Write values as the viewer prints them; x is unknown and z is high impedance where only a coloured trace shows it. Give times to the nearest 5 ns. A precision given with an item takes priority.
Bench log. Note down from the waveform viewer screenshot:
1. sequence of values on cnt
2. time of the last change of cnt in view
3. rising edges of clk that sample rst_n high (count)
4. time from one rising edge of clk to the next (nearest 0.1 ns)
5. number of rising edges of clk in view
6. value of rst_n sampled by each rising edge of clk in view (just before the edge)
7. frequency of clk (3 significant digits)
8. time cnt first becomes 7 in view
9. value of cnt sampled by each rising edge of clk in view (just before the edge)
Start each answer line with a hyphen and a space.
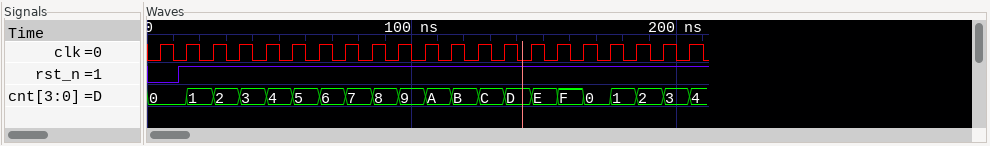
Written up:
- 0, 1, 2, 3, 4, 5, 6, 7, 8, 9, A, B, C, D, E, F, 0, 1, 2, 3, 4
- 205 ns
- 20
- 10 ns
- 21
- 0 1 1 1 1 1 1 1 1 1 1 1 1 1 1 1 1 1 1 1 1
- 100 MHz
- 75 ns
- 0, 0, 1, 2, 3, 4, 5, 6, 7, 8, 9, A, B, C, D, E, F, 0, 1, 2, 3
